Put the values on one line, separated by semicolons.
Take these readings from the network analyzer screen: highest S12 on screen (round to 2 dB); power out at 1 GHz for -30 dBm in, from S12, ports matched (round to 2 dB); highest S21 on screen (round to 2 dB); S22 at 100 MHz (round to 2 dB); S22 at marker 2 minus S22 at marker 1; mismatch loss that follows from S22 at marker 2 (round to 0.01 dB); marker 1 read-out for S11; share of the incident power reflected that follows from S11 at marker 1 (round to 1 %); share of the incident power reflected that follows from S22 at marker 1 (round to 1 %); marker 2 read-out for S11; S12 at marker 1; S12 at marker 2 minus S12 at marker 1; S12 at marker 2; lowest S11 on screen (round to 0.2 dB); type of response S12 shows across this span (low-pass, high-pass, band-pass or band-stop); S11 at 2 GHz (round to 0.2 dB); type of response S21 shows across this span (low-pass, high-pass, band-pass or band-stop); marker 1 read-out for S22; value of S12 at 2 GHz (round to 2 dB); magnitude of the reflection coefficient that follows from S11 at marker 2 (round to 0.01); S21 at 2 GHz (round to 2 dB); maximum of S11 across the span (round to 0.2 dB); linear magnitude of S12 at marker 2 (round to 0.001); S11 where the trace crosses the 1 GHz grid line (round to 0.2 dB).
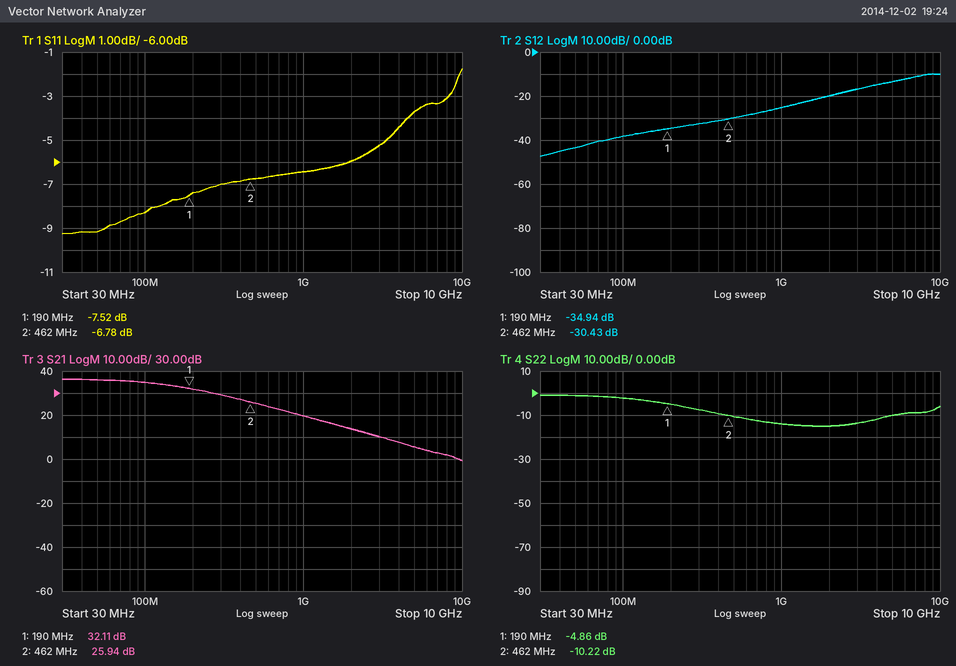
-10 dB; -56 dBm; 36 dB; -2 dB; -5.36 dB; 0.43 dB; -7.52 dB; 18 %; 33 %; -6.78 dB; -34.94 dB; 4.51 dB; -30.43 dB; -9.2 dB; high-pass; -6.0 dB; low-pass; -4.86 dB; -20 dB; 0.46; 14 dB; -1.8 dB; 0.030; -6.4 dB
